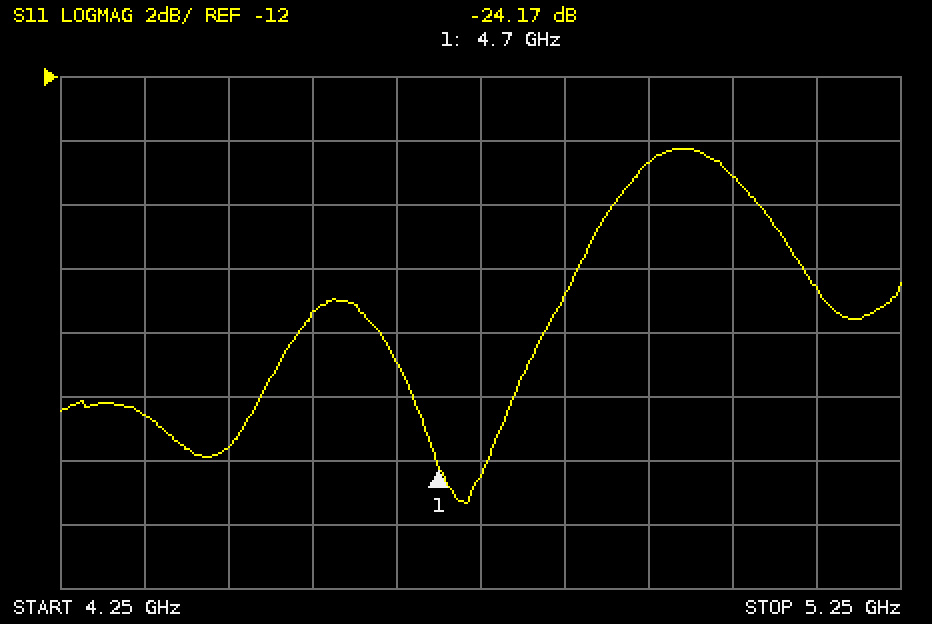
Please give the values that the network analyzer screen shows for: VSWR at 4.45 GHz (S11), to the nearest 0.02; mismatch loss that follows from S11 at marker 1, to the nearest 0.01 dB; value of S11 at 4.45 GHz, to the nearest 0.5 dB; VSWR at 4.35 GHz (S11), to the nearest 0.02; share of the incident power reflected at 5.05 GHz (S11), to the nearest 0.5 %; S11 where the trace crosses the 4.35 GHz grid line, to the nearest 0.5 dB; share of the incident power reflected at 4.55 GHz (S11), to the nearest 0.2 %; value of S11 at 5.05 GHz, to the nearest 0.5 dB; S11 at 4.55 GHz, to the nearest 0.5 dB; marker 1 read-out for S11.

1.14
0.02 dB
-23.5 dB
1.16
3.0 %
-22.5 dB
1.2 %
-15.0 dB
-19.5 dB
-24.17 dB
